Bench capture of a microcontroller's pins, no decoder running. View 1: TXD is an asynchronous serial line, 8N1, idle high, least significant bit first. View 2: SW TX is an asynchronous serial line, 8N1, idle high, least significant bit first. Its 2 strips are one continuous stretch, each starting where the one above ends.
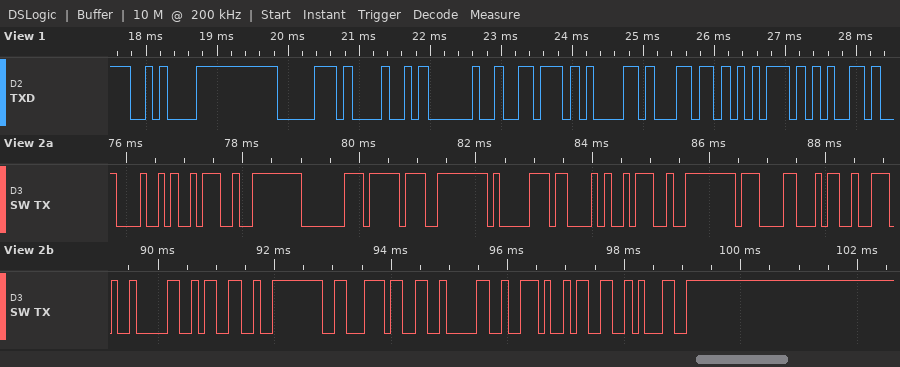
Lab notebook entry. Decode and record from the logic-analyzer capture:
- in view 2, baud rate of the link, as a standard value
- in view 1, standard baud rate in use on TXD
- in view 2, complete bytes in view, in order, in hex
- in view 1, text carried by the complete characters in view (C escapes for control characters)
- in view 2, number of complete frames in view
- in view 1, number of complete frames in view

9600 baud
9600 baud
48 3A FE C0 DF FE C1 43 3A FE 87 34 2E 30 33 FE C6 33 30 2E 33 31
"\npH value"
22
9
